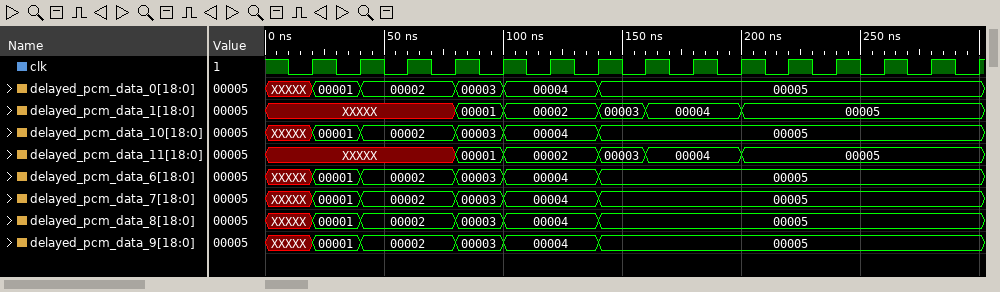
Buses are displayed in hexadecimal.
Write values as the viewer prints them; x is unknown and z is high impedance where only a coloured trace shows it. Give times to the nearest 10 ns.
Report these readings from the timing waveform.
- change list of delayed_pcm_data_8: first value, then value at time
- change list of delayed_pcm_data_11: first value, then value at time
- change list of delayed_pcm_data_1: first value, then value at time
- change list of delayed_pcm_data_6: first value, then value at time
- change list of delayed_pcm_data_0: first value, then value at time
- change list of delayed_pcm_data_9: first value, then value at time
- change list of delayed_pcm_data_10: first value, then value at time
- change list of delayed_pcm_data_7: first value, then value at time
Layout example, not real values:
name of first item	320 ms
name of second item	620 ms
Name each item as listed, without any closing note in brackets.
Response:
change list of delayed_pcm_data_8: first value, then value at time	XXXXX, 00001 at 20 ns, 00002 at 40 ns, 00003 at 80 ns, 00004 at 100 ns, 00005 at 140 ns
change list of delayed_pcm_data_11: first value, then value at time	XXXXX, 00001 at 80 ns, 00002 at 100 ns, 00003 at 140 ns, 00004 at 160 ns, 00005 at 200 ns
change list of delayed_pcm_data_1: first value, then value at time	XXXXX, 00001 at 80 ns, 00002 at 100 ns, 00003 at 140 ns, 00004 at 160 ns, 00005 at 200 ns
change list of delayed_pcm_data_6: first value, then value at time	XXXXX, 00001 at 20 ns, 00002 at 40 ns, 00003 at 80 ns, 00004 at 100 ns, 00005 at 140 ns
change list of delayed_pcm_data_0: first value, then value at time	XXXXX, 00001 at 20 ns, 00002 at 40 ns, 00003 at 80 ns, 00004 at 100 ns, 00005 at 140 ns
change list of delayed_pcm_data_9: first value, then value at time	XXXXX, 00001 at 20 ns, 00002 at 40 ns, 00003 at 80 ns, 00004 at 100 ns, 00005 at 140 ns
change list of delayed_pcm_data_10: first value, then value at time	XXXXX, 00001 at 20 ns, 00002 at 40 ns, 00003 at 80 ns, 00004 at 100 ns, 00005 at 140 ns
change list of delayed_pcm_data_7: first value, then value at time	XXXXX, 00001 at 20 ns, 00002 at 40 ns, 00003 at 80 ns, 00004 at 100 ns, 00005 at 140 ns
